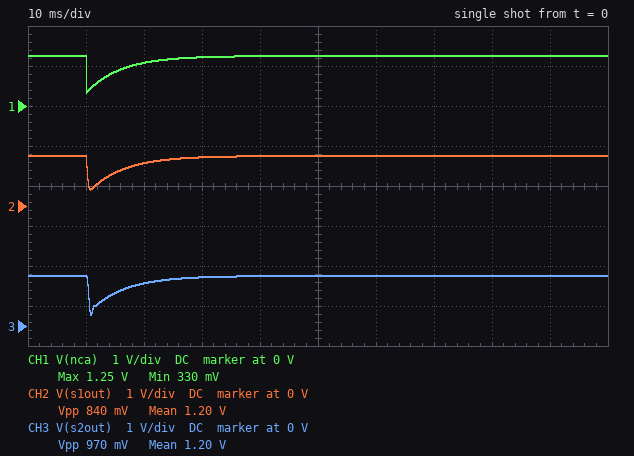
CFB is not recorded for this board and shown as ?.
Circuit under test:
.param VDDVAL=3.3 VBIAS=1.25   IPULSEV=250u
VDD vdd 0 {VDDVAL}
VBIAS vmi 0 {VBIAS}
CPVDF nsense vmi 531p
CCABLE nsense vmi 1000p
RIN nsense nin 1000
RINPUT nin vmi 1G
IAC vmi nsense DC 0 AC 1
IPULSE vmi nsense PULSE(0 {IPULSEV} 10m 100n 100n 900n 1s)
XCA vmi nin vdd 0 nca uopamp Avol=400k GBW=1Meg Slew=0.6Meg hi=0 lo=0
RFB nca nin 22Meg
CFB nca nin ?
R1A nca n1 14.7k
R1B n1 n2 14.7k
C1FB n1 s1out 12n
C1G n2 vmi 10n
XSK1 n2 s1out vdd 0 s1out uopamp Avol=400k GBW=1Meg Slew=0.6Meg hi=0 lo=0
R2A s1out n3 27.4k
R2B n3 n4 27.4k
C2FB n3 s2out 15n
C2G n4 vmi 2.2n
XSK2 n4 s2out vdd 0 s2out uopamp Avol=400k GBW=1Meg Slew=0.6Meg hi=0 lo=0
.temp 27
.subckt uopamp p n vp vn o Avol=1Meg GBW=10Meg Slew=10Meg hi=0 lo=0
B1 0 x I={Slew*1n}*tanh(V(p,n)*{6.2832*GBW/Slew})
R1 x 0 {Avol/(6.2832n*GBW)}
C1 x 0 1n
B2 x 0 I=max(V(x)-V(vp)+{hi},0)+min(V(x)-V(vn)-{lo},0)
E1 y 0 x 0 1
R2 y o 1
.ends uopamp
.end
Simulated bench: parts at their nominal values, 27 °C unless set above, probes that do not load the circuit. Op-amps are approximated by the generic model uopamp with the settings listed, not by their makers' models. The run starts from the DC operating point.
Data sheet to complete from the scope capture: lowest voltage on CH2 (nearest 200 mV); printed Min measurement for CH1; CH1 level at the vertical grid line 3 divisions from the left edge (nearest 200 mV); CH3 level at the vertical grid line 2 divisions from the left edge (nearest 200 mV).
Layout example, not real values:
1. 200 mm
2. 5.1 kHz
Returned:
1. 400 mV
2. 330 mV
3. 1.2 V
4. 1.0 V
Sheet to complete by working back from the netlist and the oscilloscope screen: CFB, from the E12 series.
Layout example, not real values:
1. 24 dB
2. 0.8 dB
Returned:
1. 270 pF
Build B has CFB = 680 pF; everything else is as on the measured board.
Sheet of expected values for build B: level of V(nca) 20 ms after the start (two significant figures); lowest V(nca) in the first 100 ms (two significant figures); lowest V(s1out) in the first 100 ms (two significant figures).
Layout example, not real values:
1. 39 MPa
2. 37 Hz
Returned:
1. 1.1 V
2. 880 mV
3. 900 mV
